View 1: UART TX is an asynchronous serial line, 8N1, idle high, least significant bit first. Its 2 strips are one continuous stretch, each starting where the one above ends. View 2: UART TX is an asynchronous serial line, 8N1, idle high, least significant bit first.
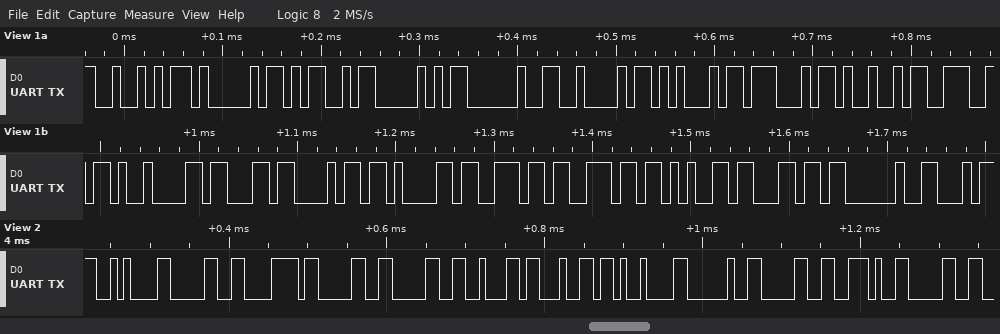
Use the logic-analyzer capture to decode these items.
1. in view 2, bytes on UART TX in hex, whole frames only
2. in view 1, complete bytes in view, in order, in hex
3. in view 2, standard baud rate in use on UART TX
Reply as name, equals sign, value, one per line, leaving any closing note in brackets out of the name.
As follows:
in view 2, bytes on UART TX in hex, whole frames only = 0x0A 0x30 0x78 0x30 0x30 0x62 0x64 0x09 0x20 0x30 0x2E 0x30
in view 1, complete bytes in view, in order, in hex = 52 41 4D 50 20 42 45 47 49 4E 09 63 68 61 6E 6E 65 6C 20
in view 2, standard baud rate in use on UART TX = 115200 baud
